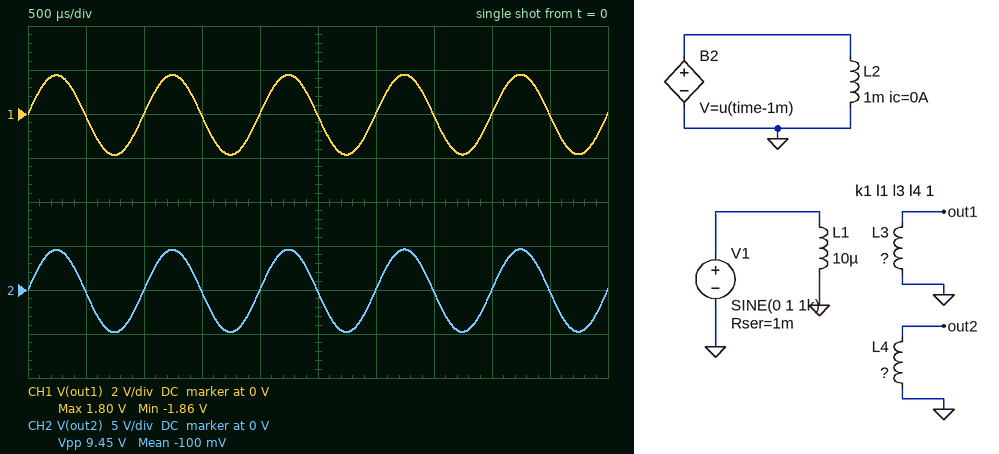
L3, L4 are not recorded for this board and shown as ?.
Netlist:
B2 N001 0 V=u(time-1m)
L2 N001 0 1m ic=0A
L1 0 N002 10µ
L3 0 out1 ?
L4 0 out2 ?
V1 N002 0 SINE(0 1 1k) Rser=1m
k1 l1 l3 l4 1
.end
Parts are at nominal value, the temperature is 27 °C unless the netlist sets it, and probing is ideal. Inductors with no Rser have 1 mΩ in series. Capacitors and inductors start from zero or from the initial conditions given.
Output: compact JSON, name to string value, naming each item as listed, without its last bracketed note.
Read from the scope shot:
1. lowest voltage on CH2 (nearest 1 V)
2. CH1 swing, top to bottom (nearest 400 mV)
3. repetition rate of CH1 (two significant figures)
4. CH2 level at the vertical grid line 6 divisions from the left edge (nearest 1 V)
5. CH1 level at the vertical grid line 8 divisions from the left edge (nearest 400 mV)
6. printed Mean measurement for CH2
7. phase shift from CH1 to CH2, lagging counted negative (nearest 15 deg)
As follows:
{"lowest voltage on CH2": "-5 V", "CH1 swing, top to bottom": "3.6 V", "repetition rate of CH1": "1.0 kHz", "CH2 level at the vertical grid line 6 divisions from the left edge": "0 V", "CH1 level at the vertical grid line 8 divisions from the left edge": "0 V", "printed Mean measurement for CH2": "-100 mV", "phase shift from CH1 to CH2, lagging counted negative": "0 deg"}
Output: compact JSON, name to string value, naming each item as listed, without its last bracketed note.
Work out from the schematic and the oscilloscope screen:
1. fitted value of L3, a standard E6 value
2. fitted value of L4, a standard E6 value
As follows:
{"fitted value of L3, a standard E6 value": "33 µH", "fitted value of L4, a standard E6 value": "220 µH"}
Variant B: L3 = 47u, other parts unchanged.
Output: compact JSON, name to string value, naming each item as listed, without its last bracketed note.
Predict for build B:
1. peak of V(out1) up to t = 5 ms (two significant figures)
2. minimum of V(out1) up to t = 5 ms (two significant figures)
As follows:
{"peak of V(out1) up to t = 5 ms": "2.1 V", "minimum of V(out1) up to t = 5 ms": "-2.2 V"}
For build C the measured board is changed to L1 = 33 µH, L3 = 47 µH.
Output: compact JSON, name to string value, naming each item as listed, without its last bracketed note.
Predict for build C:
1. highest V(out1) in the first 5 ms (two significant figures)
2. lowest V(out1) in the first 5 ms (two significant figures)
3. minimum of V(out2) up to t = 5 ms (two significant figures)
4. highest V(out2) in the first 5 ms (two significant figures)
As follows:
{"highest V(out1) in the first 5 ms": "1.2 V", "lowest V(out1) in the first 5 ms": "-1.2 V", "minimum of V(out2) up to t = 5 ms": "-2.6 V", "highest V(out2) in the first 5 ms": "2.6 V"}
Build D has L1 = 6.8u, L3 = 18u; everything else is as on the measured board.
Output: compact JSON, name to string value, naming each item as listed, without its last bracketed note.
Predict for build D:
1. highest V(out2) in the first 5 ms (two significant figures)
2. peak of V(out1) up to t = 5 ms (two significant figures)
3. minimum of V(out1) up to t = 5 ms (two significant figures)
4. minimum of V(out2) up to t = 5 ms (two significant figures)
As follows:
{"highest V(out2) in the first 5 ms": "5.6 V", "peak of V(out1) up to t = 5 ms": "1.6 V", "minimum of V(out1) up to t = 5 ms": "-1.7 V", "minimum of V(out2) up to t = 5 ms": "-5.9 V"}
